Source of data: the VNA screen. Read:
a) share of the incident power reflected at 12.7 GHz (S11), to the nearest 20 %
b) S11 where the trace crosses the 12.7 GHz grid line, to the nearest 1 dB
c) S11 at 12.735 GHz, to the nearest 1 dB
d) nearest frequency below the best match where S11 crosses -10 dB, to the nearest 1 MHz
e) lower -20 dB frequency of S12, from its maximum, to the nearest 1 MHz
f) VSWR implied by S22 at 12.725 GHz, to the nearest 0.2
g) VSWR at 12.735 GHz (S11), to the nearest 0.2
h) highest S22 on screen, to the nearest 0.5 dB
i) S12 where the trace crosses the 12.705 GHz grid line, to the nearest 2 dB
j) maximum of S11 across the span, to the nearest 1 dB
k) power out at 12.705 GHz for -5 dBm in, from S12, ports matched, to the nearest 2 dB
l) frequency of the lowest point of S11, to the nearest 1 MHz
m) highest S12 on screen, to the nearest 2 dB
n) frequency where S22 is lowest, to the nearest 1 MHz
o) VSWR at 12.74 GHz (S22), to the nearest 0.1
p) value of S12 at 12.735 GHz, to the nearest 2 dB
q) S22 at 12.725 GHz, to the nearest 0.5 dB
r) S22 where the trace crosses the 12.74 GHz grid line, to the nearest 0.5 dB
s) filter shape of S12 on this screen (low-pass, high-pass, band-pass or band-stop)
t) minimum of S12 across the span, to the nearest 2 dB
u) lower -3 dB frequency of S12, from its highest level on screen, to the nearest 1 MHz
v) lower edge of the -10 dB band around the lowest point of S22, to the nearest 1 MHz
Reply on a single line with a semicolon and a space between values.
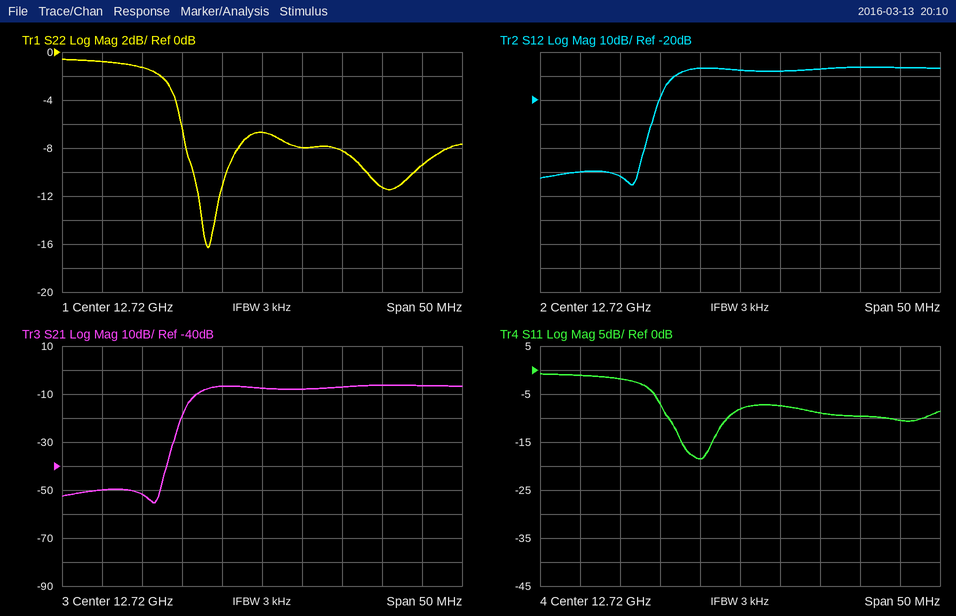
80 %; -1 dB; -10 dB; 12.711 GHz; 12.709 GHz; 2.4; 2.0; -0.5 dB; -52 dB; -1 dB; -56 dBm; 12.715 GHz; -6 dB; 12.713 GHz; 2.0; -6 dB; -8.0 dB; -9.5 dB; high-pass; -56 dB; 12.712 GHz; 12.711 GHz
